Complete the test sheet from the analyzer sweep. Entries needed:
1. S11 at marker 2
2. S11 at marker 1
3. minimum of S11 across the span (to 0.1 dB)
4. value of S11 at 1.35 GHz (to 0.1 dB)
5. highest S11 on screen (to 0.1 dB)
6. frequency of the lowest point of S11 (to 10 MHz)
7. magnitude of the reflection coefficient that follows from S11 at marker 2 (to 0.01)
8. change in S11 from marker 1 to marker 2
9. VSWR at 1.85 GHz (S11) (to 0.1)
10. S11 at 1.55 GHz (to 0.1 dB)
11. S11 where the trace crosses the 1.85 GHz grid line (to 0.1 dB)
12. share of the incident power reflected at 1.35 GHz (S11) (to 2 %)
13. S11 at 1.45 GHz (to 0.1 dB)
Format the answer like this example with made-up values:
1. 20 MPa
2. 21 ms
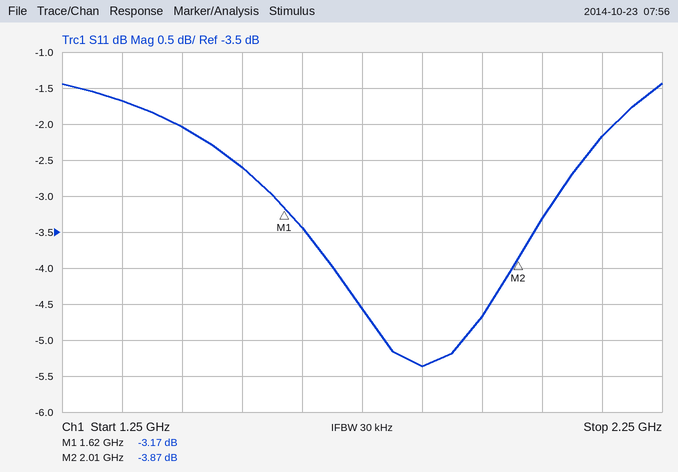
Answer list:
1. -3.87 dB
2. -3.17 dB
3. -5.4 dB
4. -1.7 dB
5. -1.4 dB
6. 1.85 GHz
7. 0.64
8. -0.70 dB
9. 3.3
10. -2.6 dB
11. -5.4 dB
12. 68 %
13. -2.0 dB
